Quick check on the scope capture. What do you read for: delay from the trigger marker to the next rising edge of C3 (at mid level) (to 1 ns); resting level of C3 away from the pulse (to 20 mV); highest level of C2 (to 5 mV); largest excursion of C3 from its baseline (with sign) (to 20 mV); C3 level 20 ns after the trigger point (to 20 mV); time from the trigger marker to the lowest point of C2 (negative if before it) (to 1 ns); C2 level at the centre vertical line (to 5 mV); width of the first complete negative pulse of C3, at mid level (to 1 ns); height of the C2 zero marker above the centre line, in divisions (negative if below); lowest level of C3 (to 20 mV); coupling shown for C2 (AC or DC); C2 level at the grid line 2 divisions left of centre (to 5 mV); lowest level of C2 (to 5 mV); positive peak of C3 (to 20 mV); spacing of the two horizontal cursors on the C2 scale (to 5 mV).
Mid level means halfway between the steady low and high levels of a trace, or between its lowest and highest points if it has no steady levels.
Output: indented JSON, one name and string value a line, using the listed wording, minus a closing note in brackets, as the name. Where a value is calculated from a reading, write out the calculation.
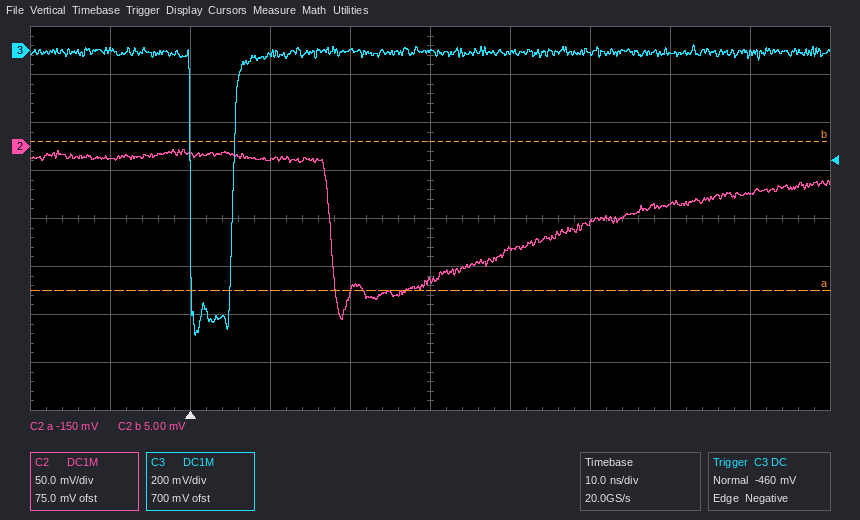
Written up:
{
  "delay from the trigger marker to the next rising edge of C3 (at mid level)": "5 ns",
  "resting level of C3 away from the pulse": "0 mV",
  "highest level of C2": "-5 mV",
  "largest excursion of C3 from its baseline (with sign)": "-1.18 V − (0 mV) = -1.18 V",
  "C3 level 20 ns after the trigger point": "0 mV",
  "time from the trigger marker to the lowest point of C2 (negative if before it)": "+19 ns",
  "C2 level at the centre vertical line": "-140 mV",
  "width of the first complete negative pulse of C3, at mid level": "5 ns",
  "height of the C2 zero marker above the centre line, in divisions": "+1.5 div",
  "lowest level of C3": "-1.18 V",
  "coupling shown for C2": "DC",
  "C2 level at the grid line 2 divisions left of centre": "-15 mV",
  "lowest level of C2": "-180 mV",
  "positive peak of C3": "20 mV",
  "spacing of the two horizontal cursors on the C2 scale": "155 mV"
}
